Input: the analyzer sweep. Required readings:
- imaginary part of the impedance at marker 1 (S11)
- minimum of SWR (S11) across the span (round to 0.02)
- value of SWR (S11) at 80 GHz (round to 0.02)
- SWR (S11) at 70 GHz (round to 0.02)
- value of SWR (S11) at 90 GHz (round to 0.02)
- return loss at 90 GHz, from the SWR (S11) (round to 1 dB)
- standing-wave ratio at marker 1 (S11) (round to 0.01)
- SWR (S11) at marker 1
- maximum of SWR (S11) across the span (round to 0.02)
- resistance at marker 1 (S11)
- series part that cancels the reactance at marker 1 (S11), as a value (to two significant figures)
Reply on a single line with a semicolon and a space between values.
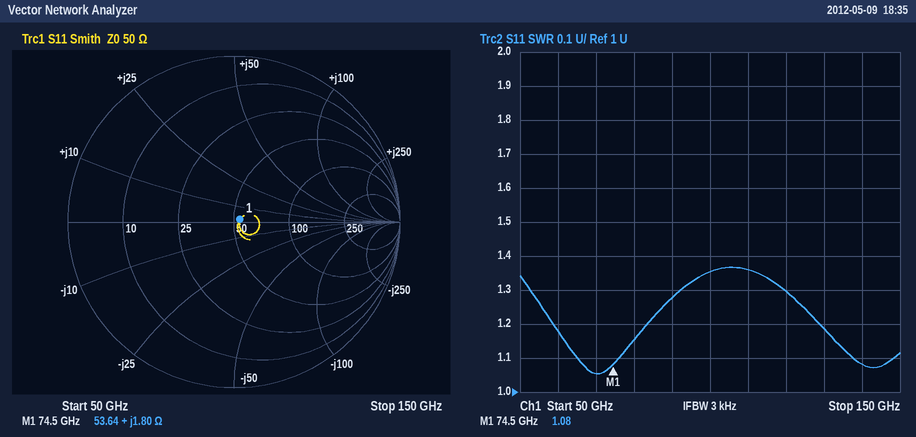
+1.80 Ω; 1.06; 1.16; 1.06; 1.28; 18 dB; 1.08; 1.08; 1.36; 53.64 Ω; 1.2 pF
